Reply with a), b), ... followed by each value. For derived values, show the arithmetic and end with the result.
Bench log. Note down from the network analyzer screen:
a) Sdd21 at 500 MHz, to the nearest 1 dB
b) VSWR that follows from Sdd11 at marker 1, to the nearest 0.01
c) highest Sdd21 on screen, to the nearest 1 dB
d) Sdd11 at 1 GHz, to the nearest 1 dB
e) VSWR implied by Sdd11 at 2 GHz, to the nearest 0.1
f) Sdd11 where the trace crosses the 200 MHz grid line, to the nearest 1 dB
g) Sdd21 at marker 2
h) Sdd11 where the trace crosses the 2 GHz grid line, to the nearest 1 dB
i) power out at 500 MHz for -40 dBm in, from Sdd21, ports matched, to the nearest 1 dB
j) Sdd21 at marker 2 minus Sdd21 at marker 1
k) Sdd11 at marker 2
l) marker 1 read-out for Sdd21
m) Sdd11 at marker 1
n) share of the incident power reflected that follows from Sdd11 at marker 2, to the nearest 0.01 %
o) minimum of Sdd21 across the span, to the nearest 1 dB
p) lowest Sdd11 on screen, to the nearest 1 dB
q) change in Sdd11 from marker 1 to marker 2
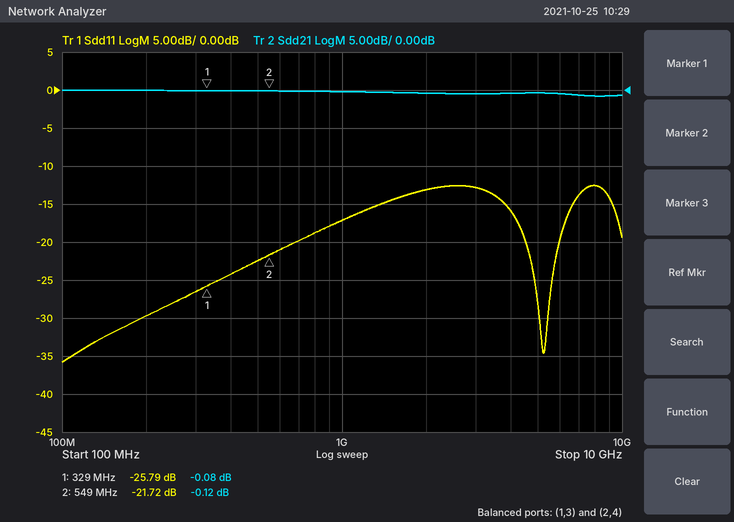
a) 0 dB
b) (1 + 0.0513)/(1 − 0.0513) ≈ 1.11
c) 0 dB
d) -17 dB
e) |Γ| = 10^(-13/20) = 0.2239; VSWR = (1 + 0.2239)/(1 − 0.2239) ≈ 1.6
f) -30 dB
g) -0.12 dB
h) -13 dB
i) -40 dBm + (0 dB) = -40 dBm
j) -0.12 − (-0.08) = -0.04 dB
k) -21.72 dB
l) -0.08 dB
m) -25.79 dB
n) 10^(-21.72/10) ≈ 0.67 %
o) -1 dB
p) -36 dB
q) -21.72 − (-25.79) = 4.07 dB
